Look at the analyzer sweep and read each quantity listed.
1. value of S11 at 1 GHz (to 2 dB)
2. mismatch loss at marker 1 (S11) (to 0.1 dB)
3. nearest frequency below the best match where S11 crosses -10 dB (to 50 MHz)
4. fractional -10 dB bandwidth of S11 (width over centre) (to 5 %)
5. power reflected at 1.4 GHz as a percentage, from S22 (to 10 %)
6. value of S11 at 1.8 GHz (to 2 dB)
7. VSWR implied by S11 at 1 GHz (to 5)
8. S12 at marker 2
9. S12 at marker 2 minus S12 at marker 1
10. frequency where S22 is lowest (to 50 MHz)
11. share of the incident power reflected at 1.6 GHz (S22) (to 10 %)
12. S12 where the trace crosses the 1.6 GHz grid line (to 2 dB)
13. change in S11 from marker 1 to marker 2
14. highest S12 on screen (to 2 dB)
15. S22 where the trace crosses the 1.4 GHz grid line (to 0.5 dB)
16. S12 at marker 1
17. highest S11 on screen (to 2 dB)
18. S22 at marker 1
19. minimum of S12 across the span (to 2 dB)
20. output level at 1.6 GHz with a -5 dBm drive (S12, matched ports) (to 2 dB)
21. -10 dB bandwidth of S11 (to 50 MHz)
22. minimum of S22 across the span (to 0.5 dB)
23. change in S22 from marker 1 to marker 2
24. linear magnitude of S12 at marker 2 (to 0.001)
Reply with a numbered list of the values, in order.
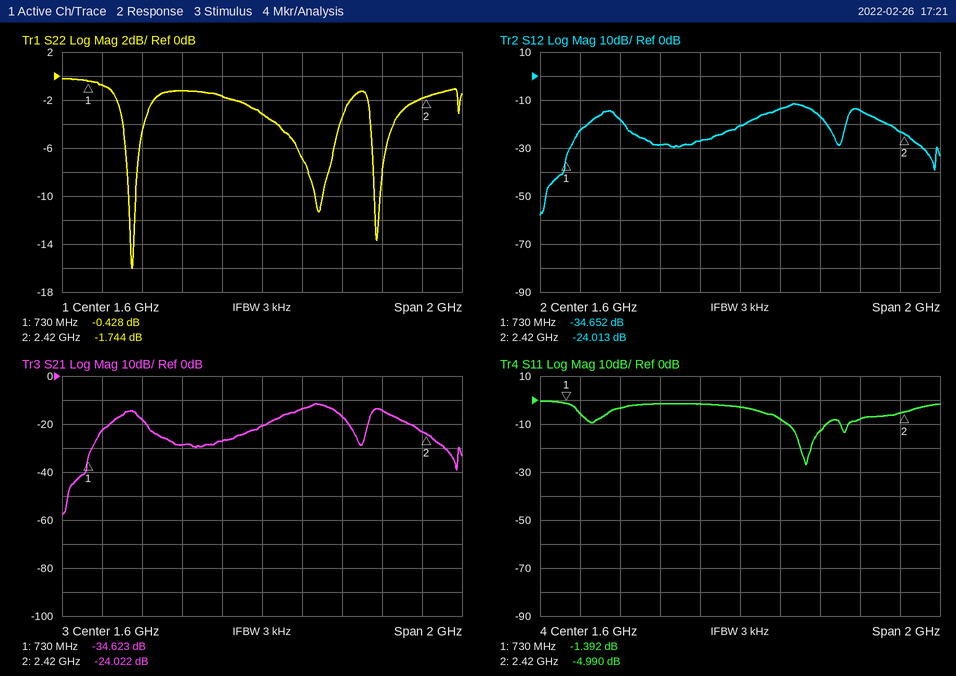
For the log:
1. -4 dB
2. 5.6 dB
3. 1.85 GHz
4. 10 %
5. 70 %
6. -8 dB
7. 5
8. -24.013 dB
9. 10.639 dB
10. 950 MHz
11. 50 %
12. -20 dB
13. -3.598 dB
14. -12 dB
15. -1.5 dB
16. -34.652 dB
17. 0 dB
18. -0.428 dB
19. -58 dB
20. -26 dBm
21. 200 MHz
22. -16.0 dB
23. -1.316 dB
24. 0.063
